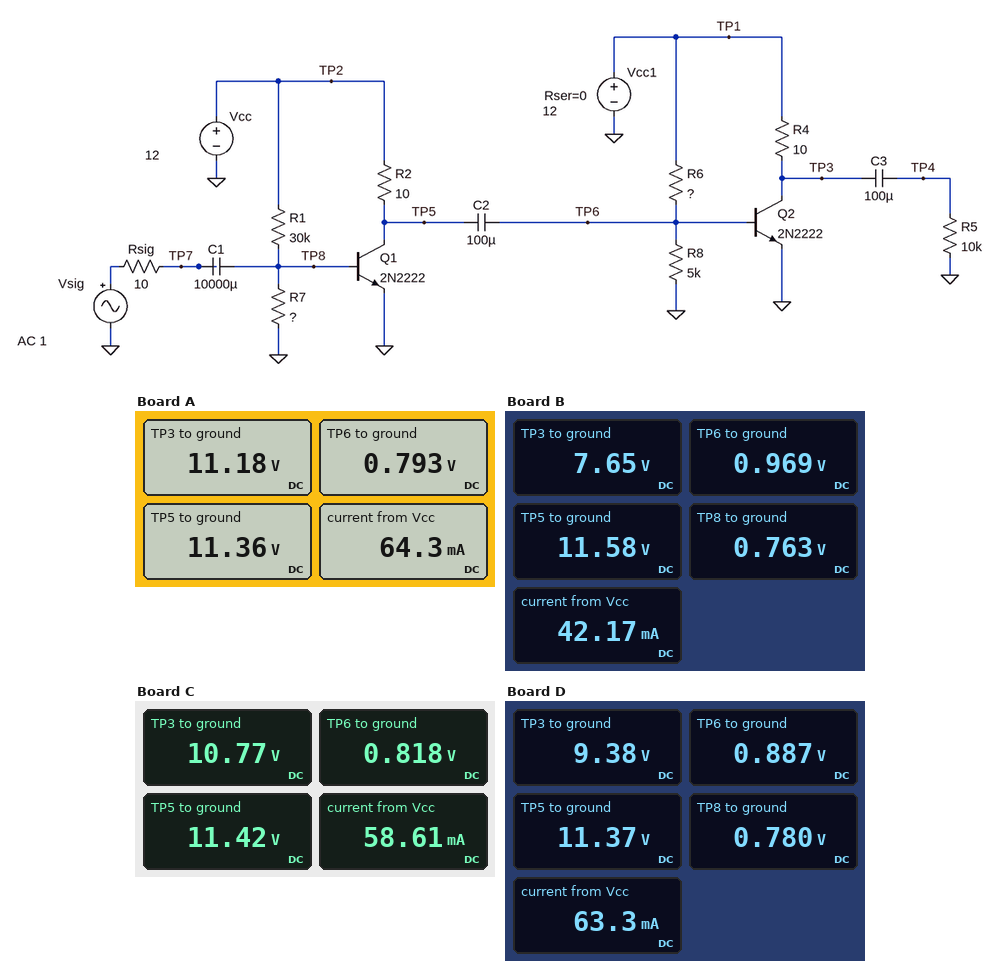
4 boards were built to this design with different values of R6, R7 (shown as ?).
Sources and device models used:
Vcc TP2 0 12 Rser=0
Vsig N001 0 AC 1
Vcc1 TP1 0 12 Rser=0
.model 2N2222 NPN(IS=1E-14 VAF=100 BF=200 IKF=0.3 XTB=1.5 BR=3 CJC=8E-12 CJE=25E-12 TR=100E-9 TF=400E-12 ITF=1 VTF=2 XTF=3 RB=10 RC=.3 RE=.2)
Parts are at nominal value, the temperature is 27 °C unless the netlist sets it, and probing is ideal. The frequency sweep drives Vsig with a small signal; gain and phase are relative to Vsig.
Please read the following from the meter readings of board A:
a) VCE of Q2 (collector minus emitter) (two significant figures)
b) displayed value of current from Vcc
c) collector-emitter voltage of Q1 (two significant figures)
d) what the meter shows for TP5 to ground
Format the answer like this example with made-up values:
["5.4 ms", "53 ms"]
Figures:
["11 V", "64.3 mA", "11 V", "11.36 V"]
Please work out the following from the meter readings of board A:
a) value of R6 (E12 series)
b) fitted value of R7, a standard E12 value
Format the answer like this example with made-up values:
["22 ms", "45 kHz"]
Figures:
["18 kΩ", "27 kΩ"]
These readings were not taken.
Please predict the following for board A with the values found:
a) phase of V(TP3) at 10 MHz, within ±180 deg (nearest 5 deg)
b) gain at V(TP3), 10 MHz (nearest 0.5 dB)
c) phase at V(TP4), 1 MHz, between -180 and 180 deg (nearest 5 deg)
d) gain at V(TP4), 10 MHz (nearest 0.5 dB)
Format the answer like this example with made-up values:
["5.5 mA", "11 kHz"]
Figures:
["-75 deg", "41.0 dB", "-10 deg", "41.0 dB"]
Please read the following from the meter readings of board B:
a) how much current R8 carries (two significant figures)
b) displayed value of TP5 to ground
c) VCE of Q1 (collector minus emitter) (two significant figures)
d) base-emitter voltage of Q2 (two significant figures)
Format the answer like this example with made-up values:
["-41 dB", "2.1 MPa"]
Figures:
["190 µA", "11.58 V", "12 V", "970 mV"]
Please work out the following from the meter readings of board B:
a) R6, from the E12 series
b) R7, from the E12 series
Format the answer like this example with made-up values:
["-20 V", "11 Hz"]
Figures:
["2.2 kΩ", "4.7 kΩ"]
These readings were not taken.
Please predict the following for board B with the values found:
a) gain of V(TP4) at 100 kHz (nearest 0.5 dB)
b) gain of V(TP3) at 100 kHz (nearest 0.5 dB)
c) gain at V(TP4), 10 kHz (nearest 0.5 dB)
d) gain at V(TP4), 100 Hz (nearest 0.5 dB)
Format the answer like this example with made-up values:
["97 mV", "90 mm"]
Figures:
["43.5 dB", "43.5 dB", "43.5 dB", "42.5 dB"]
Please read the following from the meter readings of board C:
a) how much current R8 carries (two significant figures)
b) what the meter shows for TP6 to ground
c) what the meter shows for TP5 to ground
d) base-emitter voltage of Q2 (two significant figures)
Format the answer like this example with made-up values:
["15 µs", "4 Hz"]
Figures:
["160 µA", "0.818 V", "11.42 V", "820 mV"]
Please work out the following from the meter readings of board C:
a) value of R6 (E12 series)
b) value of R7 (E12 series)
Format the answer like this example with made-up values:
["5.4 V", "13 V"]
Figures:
["12 kΩ", "12 kΩ"]
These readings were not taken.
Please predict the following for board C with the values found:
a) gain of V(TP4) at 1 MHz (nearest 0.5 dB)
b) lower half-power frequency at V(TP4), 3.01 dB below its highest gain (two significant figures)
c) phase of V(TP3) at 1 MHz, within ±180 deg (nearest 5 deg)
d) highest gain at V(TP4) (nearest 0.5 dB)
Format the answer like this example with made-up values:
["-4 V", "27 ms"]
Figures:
["45.5 dB", "21 Hz", "-10 deg", "45.5 dB"]
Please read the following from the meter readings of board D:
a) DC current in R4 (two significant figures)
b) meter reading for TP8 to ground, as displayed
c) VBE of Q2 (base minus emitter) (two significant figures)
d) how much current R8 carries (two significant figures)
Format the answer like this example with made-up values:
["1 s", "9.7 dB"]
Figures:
["260 mA", "0.780 V", "890 mV", "180 µA"]
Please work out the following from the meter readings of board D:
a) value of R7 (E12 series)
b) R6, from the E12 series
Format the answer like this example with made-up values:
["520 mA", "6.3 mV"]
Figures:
["22 kΩ", "4.7 kΩ"]
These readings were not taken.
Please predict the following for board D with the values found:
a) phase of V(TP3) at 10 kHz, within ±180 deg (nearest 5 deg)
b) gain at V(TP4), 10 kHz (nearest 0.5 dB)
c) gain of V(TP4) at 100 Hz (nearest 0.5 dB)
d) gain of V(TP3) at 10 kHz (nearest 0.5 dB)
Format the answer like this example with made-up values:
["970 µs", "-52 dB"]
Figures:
["0 deg", "46.5 dB", "46.0 dB", "46.5 dB"]
